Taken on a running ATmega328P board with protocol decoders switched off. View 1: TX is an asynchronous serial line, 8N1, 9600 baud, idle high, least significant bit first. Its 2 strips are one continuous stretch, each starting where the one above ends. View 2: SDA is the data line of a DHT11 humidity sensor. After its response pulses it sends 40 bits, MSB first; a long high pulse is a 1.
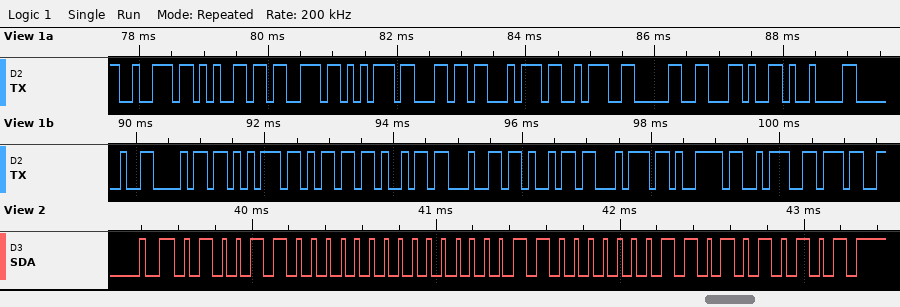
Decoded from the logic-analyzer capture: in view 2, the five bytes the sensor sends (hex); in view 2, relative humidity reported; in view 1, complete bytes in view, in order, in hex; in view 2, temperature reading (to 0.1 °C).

4C 00 06 03 55
76 %
72 65 73 75 6C 74 3A 30 2C 09 20 68 75 6D 69 64 69 74 79 3A 37
6.3 °C
